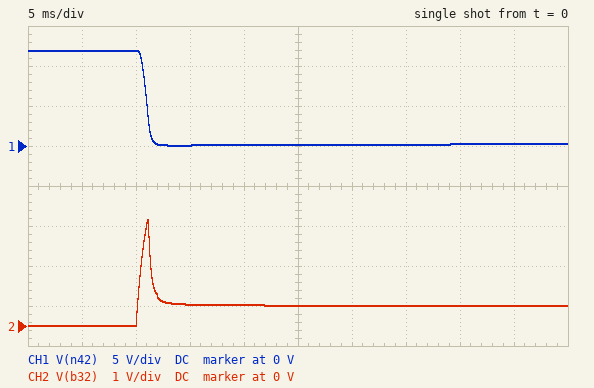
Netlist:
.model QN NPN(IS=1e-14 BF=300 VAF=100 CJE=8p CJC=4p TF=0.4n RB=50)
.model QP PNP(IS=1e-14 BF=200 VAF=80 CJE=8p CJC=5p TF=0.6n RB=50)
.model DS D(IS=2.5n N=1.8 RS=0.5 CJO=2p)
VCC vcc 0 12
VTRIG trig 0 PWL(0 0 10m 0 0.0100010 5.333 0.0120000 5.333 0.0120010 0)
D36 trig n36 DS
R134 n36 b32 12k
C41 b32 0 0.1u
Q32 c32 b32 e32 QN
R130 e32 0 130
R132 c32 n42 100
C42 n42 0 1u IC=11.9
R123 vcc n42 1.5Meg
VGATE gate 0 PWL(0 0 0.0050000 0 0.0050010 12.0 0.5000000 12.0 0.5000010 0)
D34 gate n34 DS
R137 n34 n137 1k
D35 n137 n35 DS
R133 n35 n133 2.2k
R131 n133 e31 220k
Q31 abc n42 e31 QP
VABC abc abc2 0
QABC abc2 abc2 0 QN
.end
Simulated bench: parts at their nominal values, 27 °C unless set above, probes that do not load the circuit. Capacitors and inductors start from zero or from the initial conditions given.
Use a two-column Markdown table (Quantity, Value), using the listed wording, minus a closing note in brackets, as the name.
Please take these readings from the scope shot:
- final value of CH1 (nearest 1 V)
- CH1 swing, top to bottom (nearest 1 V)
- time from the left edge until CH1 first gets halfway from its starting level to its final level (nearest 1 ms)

| Quantity | Value |
|---|---|
| final value of CH1 | 0 V |
| CH1 swing, top to bottom | 12 V |
| time from the left edge until CH1 first gets halfway from its starting level to its final level | 11 ms |
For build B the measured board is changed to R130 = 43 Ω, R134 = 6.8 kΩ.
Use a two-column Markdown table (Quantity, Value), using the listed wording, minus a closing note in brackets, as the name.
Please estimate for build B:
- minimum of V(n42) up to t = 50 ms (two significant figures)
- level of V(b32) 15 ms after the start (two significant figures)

| Quantity | Value |
|---|---|
| minimum of V(n42) up to t = 50 ms | 39 mV |
| level of V(b32) 15 ms after the start | 520 mV |
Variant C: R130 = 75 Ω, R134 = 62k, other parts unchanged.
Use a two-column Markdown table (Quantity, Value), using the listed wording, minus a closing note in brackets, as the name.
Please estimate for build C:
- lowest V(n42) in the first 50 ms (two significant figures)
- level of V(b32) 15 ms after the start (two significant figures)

| Quantity | Value |
|---|---|
| lowest V(n42) in the first 50 ms | 56 mV |
| level of V(b32) 15 ms after the start | 560 mV |
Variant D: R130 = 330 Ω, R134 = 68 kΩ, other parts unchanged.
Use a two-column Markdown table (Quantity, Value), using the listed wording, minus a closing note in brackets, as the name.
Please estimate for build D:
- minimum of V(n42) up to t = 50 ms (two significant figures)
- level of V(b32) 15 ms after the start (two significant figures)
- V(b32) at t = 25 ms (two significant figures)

| Quantity | Value |
|---|---|
| minimum of V(n42) up to t = 50 ms | 64 mV |
| level of V(b32) 15 ms after the start | 1.1 V |
| V(b32) at t = 25 ms | 550 mV |
